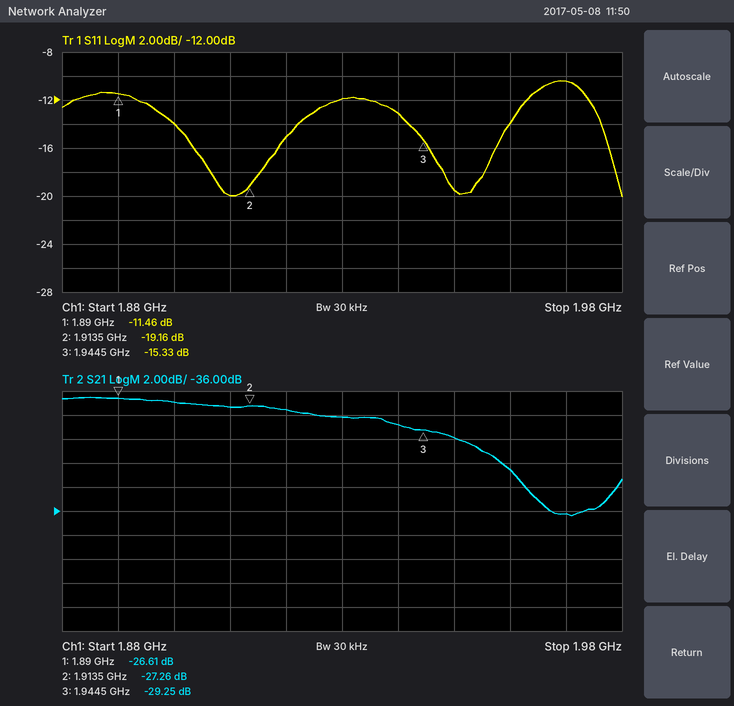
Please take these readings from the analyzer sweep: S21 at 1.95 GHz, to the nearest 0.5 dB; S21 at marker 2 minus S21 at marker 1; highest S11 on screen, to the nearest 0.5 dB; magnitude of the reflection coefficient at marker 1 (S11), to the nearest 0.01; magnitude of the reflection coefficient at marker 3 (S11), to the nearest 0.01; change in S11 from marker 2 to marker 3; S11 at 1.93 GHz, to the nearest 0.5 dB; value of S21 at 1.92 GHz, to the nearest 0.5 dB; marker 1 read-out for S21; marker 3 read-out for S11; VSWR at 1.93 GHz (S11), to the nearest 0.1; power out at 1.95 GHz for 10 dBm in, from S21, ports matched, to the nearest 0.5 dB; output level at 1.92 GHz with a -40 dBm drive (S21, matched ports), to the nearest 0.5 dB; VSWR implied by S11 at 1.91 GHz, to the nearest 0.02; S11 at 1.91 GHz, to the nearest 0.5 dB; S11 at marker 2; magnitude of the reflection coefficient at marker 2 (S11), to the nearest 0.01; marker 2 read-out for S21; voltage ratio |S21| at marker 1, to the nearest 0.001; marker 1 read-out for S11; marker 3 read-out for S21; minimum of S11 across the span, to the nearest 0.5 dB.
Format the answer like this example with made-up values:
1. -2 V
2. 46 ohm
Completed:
1. -30.0 dB
2. -0.65 dB
3. -10.5 dB
4. 0.27
5. 0.17
6. 3.83 dB
7. -12.0 dB
8. -27.5 dB
9. -26.61 dB
10. -15.33 dB
11. 1.7
12. -20.0 dBm
13. -67.5 dBm
14. 1.22
15. -20.0 dB
16. -19.16 dB
17. 0.11
18. -27.26 dB
19. 0.047
20. -11.46 dB
21. -29.25 dB
22. -20.0 dB
